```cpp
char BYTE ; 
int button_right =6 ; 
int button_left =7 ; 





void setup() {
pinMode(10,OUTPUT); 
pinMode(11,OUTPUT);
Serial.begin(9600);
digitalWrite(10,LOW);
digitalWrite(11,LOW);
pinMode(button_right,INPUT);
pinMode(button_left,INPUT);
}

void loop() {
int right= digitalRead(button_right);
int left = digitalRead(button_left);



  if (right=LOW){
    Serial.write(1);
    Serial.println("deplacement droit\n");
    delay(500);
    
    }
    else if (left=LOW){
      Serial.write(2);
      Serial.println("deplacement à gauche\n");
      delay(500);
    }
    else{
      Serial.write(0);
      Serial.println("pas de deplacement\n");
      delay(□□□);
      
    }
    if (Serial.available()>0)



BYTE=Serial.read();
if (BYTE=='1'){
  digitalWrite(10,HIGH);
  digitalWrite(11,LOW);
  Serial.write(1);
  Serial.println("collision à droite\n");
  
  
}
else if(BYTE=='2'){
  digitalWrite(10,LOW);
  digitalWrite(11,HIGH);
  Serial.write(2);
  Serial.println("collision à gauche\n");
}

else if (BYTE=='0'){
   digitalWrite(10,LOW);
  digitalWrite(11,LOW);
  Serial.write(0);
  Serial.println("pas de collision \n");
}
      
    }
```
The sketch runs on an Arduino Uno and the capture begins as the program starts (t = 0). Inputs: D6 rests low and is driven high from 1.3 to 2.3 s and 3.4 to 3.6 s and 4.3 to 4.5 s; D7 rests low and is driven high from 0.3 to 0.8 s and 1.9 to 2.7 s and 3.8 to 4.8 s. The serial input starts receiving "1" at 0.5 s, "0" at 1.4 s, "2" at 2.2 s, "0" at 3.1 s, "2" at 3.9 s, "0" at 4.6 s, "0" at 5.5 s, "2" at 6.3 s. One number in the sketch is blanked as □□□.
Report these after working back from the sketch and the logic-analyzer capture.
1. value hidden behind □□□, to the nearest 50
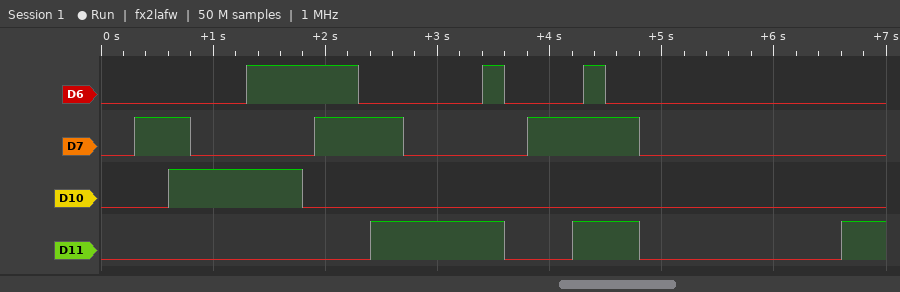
600
